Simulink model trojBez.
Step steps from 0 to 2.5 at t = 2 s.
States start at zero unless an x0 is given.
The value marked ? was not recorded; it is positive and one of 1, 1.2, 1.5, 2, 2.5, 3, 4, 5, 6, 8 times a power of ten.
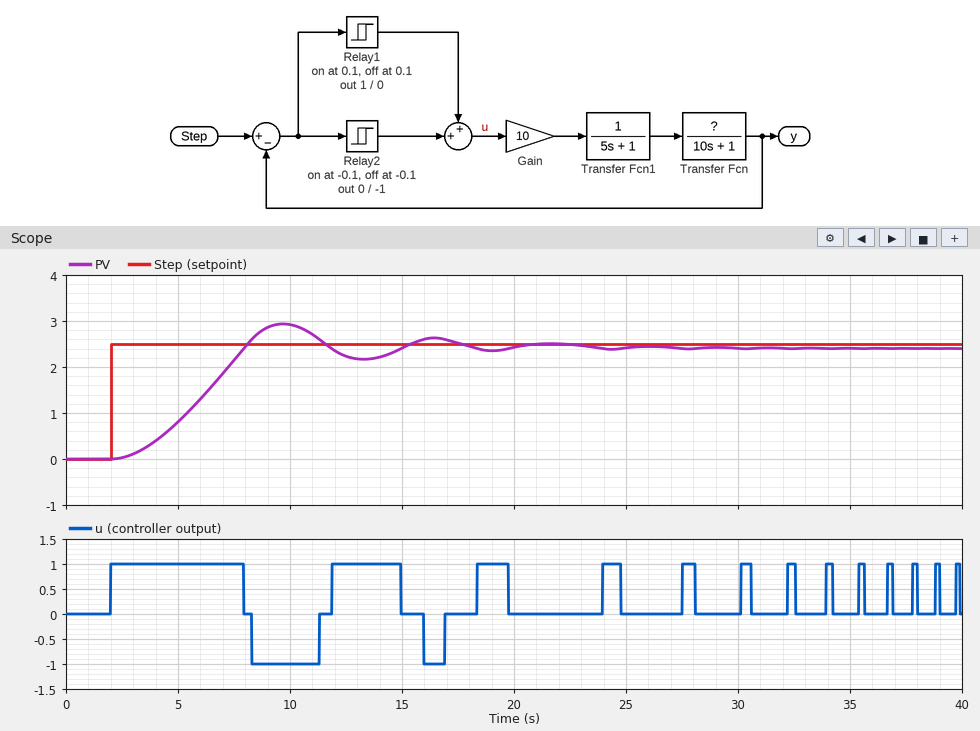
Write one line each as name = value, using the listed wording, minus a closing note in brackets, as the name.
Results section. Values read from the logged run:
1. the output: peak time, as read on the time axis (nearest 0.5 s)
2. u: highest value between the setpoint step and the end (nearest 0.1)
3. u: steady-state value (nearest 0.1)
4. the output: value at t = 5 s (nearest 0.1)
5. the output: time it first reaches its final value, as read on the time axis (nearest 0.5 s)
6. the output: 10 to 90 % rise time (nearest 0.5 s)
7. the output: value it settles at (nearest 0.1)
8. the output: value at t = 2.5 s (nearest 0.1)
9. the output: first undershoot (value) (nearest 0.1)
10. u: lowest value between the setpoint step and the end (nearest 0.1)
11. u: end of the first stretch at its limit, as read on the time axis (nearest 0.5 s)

the output: peak time, as read on the time axis = 9.5 s
u: highest value between the setpoint step and the end = 1.0
u: steady-state value = 0.0
the output: value at t = 5 s = 0.8
the output: time it first reaches its final value, as read on the time axis = 8.0 s
the output: 10 to 90 % rise time = 4.0 s
the output: value it settles at = 2.4
the output: value at t = 2.5 s = 0.0
the output: first undershoot (value) = 2.2
u: lowest value between the setpoint step and the end = -1.0
u: end of the first stretch at its limit, as read on the time axis = 8.0 s
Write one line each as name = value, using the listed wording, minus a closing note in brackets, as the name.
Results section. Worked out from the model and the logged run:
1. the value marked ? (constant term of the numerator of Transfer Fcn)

the value marked ? = 1.2
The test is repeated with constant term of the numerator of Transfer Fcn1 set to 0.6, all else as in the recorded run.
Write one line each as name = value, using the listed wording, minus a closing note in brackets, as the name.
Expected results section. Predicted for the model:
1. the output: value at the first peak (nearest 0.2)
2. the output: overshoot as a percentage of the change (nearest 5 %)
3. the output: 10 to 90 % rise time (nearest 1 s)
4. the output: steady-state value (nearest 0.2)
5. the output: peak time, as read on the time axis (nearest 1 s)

the output: value at the first peak = 2.8
the output: overshoot as a percentage of the change = 15 %
the output: 10 to 90 % rise time = 6 s
the output: steady-state value = 2.4
the output: peak time, as read on the time axis = 12 s
